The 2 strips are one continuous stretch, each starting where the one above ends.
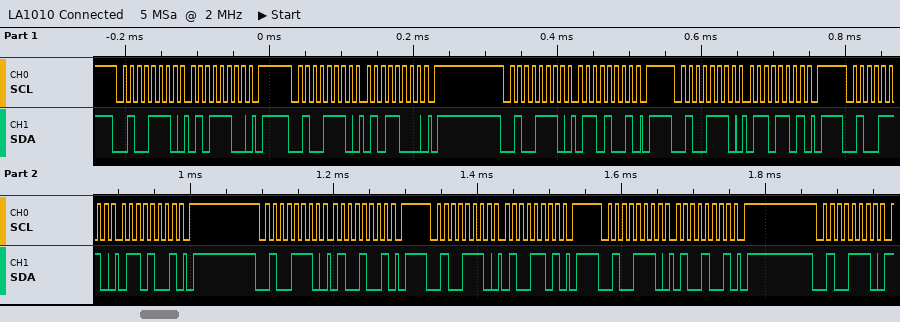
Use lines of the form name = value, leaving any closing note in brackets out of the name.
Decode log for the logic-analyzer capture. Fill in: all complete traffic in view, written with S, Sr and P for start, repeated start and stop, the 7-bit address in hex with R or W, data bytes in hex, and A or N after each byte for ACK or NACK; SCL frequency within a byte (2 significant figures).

all complete traffic in view, written with S, Sr and P for start, repeated start and stop, the 7-bit address in hex with R or W, data bytes in hex, and A or N after each byte for ACK or NACK = S 27W A 5C A P S 27W A 58 A P S 27W A 69 A P S 27W A 6D A P S 27W A 69 A P S 27W A 49 A P S 27W A 4D A P S 27W A 49 A P S 27W A
SCL frequency within a byte = 100 kHz
